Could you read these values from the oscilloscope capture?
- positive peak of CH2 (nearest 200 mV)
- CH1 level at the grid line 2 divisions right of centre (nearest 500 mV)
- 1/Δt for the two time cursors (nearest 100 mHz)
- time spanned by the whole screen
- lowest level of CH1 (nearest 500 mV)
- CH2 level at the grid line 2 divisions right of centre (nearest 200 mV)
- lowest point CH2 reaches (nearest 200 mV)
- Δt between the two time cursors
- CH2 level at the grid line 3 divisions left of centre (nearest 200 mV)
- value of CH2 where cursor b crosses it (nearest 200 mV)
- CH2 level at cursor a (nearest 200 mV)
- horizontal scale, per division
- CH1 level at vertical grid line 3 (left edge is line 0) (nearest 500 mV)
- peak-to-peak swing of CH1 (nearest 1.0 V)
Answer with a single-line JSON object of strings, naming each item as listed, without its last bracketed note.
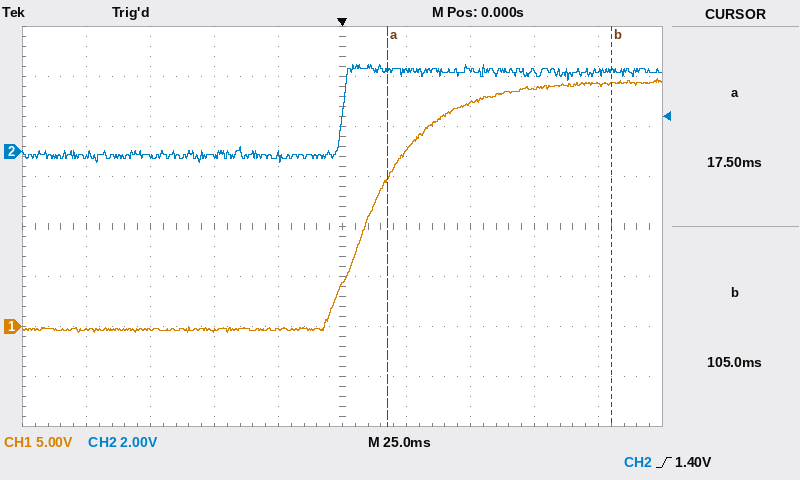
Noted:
{"positive peak of CH2": "3.4 V", "CH1 level at the grid line 2 divisions right of centre": "22.5 V", "1/Δt for the two time cursors": "11.4 Hz", "time spanned by the whole screen": "250 ms", "lowest level of CH1": "-500 mV", "CH2 level at the grid line 2 divisions right of centre": "3.2 V", "lowest point CH2 reaches": "-400 mV", "Δt between the two time cursors": "87.5 ms", "CH2 level at the grid line 3 divisions left of centre": "-200 mV", "value of CH2 where cursor b crosses it": "3.2 V", "CH2 level at cursor a": "3.2 V", "horizontal scale, per division": "25 ms", "CH1 level at vertical grid line 3 (left edge is line 0)": "-500 mV", "peak-to-peak swing of CH1": "25.0 V"}
